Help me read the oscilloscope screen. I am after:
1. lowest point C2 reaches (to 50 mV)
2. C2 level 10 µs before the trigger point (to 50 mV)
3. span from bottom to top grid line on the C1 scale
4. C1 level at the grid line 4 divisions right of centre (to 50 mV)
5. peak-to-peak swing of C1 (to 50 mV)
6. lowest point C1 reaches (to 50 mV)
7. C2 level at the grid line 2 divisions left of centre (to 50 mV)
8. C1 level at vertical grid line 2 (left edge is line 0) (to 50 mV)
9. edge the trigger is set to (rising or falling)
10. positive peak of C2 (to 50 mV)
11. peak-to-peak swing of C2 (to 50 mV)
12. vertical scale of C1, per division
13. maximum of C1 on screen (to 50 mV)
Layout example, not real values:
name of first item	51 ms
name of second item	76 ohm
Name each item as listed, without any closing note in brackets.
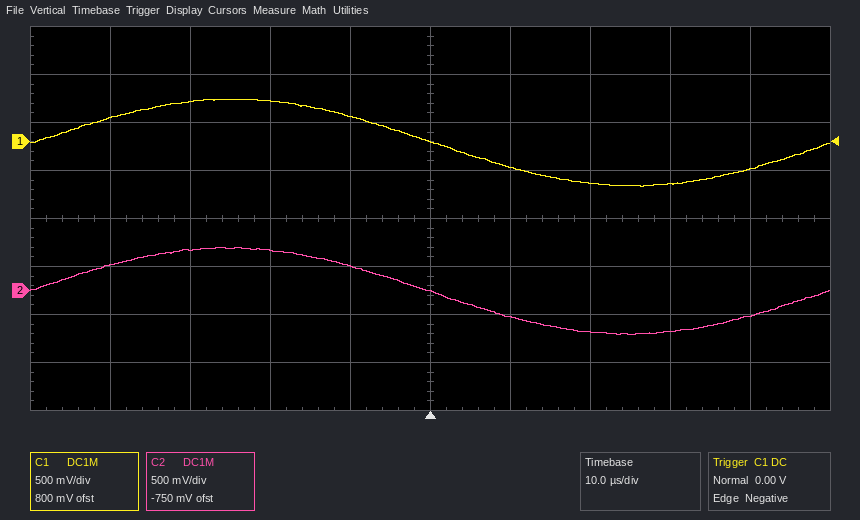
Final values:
lowest point C2 reaches	-450 mV
C2 level 10 µs before the trigger point	250 mV
span from bottom to top grid line on the C1 scale	4 V
C1 level at the grid line 4 divisions right of centre	-300 mV
peak-to-peak swing of C1	900 mV
lowest point C1 reaches	-450 mV
C2 level at the grid line 2 divisions left of centre	400 mV
C1 level at vertical grid line 2 (left edge is line 0)	400 mV
edge the trigger is set to	falling
positive peak of C2	450 mV
peak-to-peak swing of C2	900 mV
vertical scale of C1, per division	500 mV
maximum of C1 on screen	450 mV
